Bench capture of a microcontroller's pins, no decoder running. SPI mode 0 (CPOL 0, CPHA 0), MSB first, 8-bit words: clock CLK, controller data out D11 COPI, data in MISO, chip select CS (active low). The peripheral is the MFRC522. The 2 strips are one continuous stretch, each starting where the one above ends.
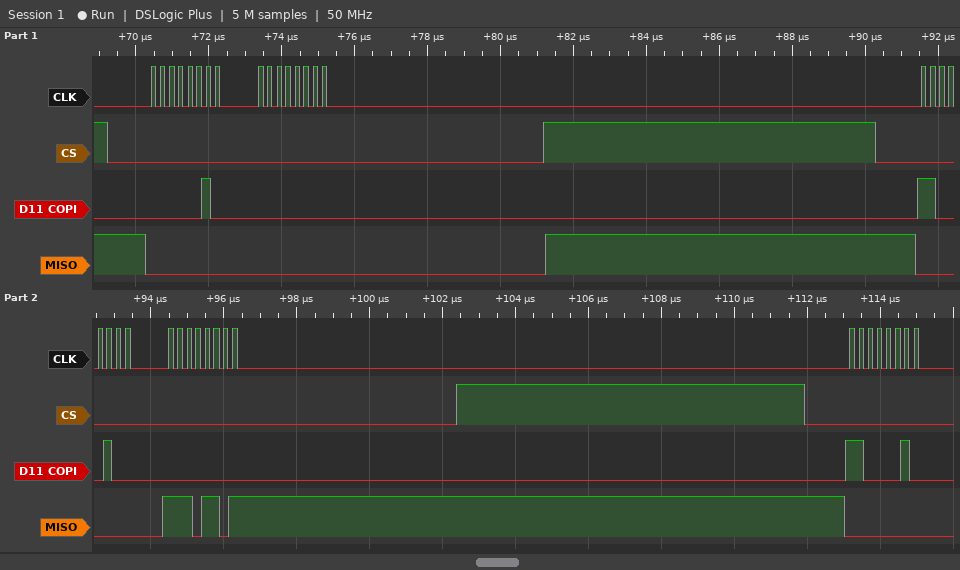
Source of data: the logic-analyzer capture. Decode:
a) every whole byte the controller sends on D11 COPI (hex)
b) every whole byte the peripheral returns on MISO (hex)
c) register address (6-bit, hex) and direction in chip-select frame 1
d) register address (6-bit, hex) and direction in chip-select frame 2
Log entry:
02 00 C4 00 C2
00 00 00 ED 00
0x01 write
0x22 read
